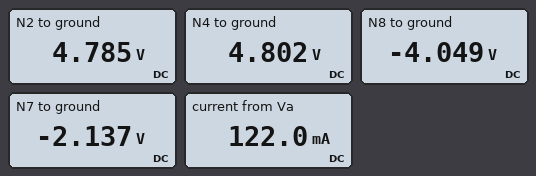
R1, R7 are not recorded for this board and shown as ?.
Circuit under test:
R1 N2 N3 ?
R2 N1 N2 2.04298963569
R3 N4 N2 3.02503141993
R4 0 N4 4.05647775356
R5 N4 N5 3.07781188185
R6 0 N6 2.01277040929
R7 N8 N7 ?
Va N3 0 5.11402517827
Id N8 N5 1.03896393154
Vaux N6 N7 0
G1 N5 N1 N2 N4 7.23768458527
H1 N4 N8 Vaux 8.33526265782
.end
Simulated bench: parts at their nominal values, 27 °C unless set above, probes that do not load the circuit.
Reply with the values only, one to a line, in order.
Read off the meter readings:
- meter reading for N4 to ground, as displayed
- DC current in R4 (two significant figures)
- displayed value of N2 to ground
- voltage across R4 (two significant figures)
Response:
4.802 V
1.2 A
4.785 V
4.8 V
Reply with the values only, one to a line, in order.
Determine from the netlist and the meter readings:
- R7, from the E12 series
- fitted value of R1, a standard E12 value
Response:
1.8 Ω
2.7 Ω
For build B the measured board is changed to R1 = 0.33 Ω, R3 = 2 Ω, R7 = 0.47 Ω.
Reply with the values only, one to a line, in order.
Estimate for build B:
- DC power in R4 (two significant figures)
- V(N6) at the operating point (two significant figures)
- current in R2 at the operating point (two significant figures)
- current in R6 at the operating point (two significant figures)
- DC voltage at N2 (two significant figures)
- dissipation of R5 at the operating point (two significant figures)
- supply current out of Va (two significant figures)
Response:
6.3 W
-1.7 V
410 mA
860 mA
5.0 V
6.5 W
380 mA
